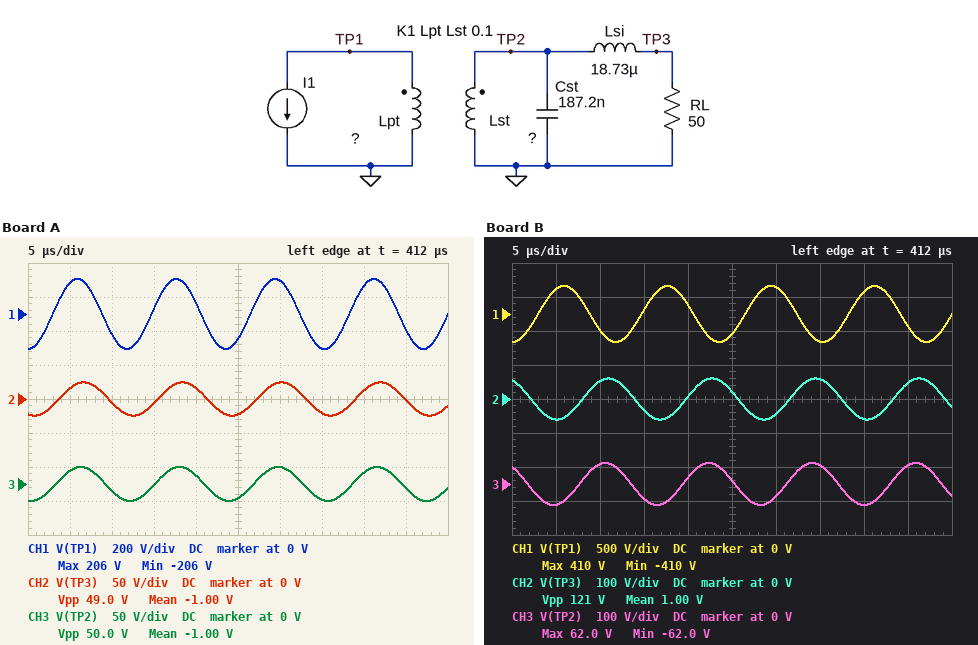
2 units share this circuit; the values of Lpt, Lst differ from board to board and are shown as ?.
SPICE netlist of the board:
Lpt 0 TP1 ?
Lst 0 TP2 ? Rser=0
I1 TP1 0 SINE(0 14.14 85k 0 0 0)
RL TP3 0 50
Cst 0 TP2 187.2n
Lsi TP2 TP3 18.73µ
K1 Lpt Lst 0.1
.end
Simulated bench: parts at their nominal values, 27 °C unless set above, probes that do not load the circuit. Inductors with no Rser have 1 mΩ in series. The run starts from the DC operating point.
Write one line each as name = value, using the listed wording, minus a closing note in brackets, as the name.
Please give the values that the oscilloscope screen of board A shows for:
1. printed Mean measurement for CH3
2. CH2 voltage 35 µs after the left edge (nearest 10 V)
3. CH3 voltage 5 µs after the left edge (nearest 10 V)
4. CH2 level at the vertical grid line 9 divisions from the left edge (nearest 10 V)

printed Mean measurement for CH3 = -1.00 V
CH2 voltage 35 µs after the left edge = -20 V
CH3 voltage 5 µs after the left edge = 20 V
CH2 level at the vertical grid line 9 divisions from the left edge = 0 V
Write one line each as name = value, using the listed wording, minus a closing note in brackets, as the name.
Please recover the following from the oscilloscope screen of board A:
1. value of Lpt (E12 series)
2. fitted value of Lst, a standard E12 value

value of Lpt = 27 µH
fitted value of Lst, a standard E12 value = 10 µH
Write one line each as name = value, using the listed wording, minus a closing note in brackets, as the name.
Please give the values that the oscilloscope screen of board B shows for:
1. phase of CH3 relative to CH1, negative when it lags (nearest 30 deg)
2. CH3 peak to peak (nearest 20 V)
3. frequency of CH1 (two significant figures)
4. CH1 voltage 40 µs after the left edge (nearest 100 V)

phase of CH3 relative to CH1, negative when it lags = -150 deg
CH3 peak to peak = 120 V
frequency of CH1 = 85 kHz
CH1 voltage 40 µs after the left edge = 300 V
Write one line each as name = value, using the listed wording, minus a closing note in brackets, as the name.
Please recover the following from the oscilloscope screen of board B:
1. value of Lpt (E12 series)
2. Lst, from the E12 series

value of Lpt = 56 µH
Lst, from the E12 series = 27 µH
